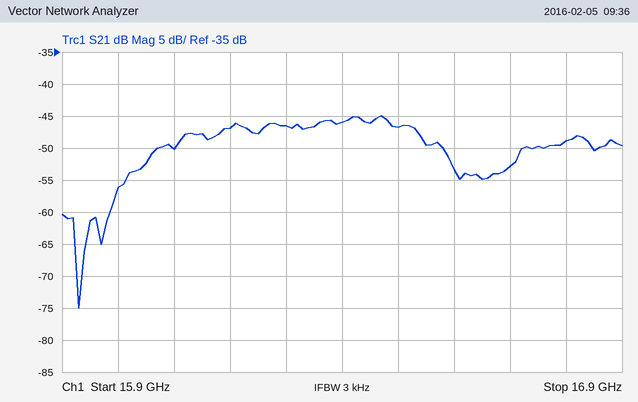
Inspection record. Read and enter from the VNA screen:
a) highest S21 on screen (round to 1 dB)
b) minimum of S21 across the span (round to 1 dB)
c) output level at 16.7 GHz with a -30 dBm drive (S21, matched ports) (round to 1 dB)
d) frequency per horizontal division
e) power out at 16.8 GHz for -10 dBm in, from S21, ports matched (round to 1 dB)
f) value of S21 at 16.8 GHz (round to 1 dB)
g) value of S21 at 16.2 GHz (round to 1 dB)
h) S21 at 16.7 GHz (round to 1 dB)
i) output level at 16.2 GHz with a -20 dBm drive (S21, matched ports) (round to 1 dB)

-45 dB
-75 dB
-83 dBm
100 MHz
-59 dBm
-49 dB
-47 dB
-53 dB
-67 dBm
